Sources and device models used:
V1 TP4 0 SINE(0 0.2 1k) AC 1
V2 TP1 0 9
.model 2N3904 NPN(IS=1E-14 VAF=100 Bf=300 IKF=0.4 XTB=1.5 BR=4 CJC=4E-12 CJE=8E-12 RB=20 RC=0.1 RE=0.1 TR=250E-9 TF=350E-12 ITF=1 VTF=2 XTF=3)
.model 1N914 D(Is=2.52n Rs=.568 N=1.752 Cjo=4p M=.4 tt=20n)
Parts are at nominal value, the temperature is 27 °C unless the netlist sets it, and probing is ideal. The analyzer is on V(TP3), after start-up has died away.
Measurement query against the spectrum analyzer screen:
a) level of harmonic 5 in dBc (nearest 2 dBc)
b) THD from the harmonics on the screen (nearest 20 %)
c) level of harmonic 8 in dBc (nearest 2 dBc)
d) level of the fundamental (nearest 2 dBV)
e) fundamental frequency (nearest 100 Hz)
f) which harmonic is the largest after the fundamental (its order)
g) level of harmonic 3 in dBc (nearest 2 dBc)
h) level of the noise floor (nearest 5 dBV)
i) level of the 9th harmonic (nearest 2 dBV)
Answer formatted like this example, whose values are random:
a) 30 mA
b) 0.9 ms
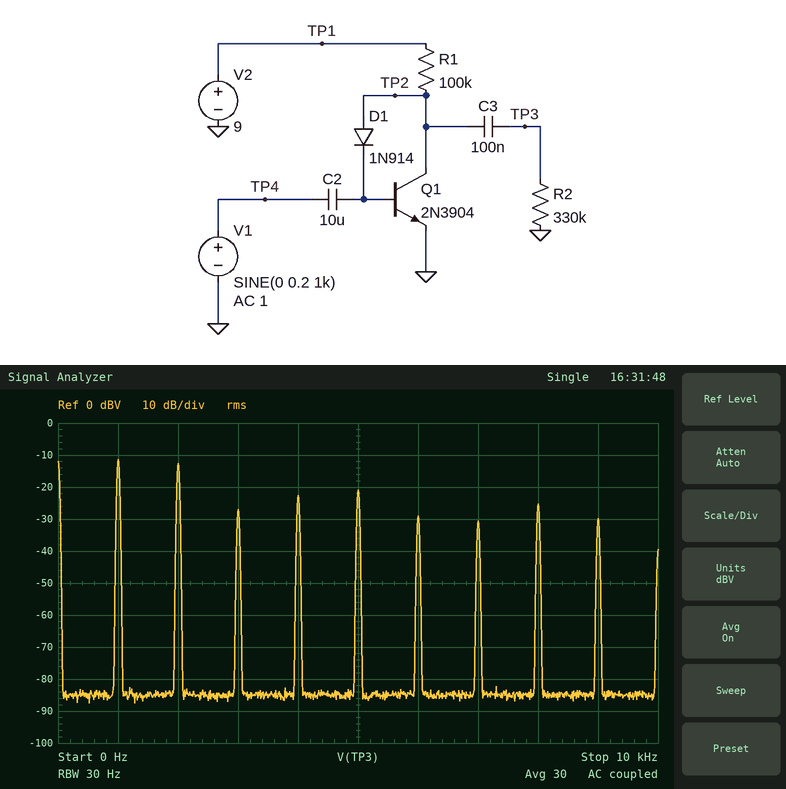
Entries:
a) -10 dBc
b) 100 %
c) -14 dBc
d) -12 dBV
e) 1.0 kHz
f) 2
g) -16 dBc
h) -85 dBV
i) -30 dBV
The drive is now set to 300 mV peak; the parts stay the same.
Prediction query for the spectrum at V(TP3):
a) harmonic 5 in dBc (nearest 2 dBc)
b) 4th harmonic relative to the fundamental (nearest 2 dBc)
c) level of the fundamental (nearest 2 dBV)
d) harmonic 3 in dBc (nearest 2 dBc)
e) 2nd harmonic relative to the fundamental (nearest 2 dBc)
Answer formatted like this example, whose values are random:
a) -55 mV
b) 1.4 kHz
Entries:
a) -6 dBc
b) -22 dBc
c) -16 dBV
d) -4 dBc
e) 4 dBc
